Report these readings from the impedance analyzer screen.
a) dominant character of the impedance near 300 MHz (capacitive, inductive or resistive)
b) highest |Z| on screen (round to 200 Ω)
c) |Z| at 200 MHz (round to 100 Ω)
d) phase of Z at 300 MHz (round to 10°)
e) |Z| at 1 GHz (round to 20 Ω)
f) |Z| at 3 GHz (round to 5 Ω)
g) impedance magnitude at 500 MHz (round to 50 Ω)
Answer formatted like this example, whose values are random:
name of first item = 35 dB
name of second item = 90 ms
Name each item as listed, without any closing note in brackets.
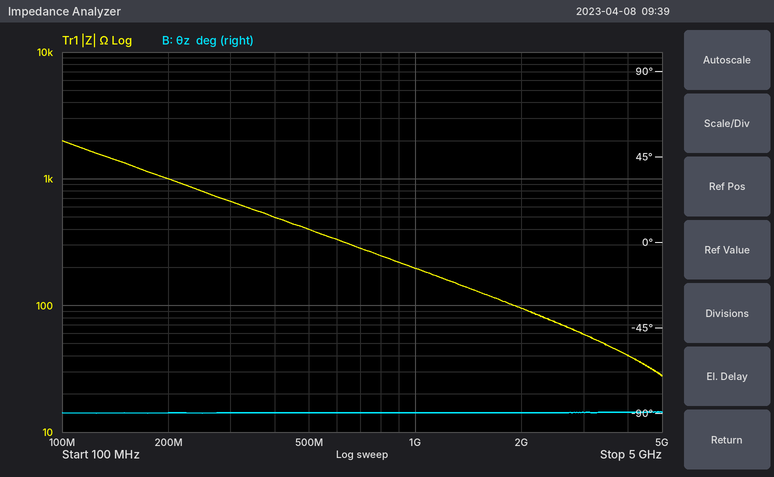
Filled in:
dominant character of the impedance near 300 MHz = capacitive
highest |Z| on screen = 2.0 kΩ
|Z| at 200 MHz = 1.0 kΩ
phase of Z at 300 MHz = -90°
|Z| at 1 GHz = 200 Ω
|Z| at 3 GHz = 60 Ω
impedance magnitude at 500 MHz = 400 Ω
